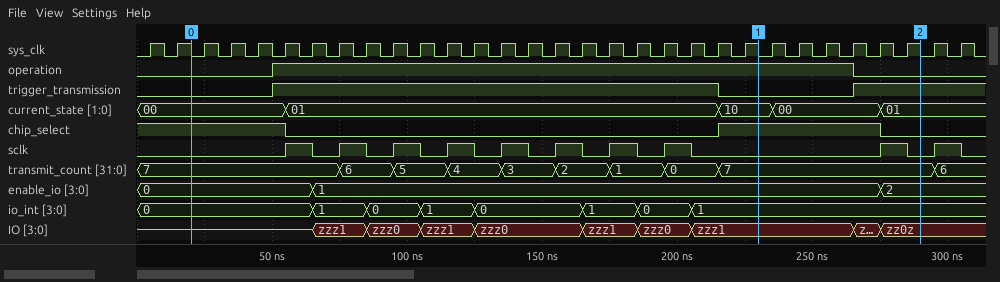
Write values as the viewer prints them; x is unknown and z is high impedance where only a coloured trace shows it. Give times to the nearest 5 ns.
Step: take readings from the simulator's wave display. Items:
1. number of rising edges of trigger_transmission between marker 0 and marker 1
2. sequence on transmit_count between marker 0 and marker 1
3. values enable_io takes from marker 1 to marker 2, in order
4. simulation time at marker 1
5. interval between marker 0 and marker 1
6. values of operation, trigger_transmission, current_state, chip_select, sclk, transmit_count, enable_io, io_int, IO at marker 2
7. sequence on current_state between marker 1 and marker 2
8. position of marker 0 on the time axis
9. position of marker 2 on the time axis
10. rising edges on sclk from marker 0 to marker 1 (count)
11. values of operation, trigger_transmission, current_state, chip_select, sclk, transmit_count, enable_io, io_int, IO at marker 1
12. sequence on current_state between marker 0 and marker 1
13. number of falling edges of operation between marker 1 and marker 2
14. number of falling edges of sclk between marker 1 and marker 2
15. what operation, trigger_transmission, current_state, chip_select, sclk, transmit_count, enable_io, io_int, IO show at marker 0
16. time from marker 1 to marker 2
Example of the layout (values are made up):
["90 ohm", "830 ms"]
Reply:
["1", "7, 6, 5, 4, 3, 2, 1, 0, 7", "1, 2", "230 ns", "210 ns", "operation=0, trigger_transmission=1, current_state=01, chip_select=0, sclk=0, transmit_count=7, enable_io=2, io_int=1, IO=zz0z", "10, 00, 01", "20 ns", "290 ns", "8", "operation=1, trigger_transmission=0, current_state=10, chip_select=1, sclk=0, transmit_count=7, enable_io=1, io_int=1, IO=zzz1", "00, 01, 10", "1", "1", "operation=0, trigger_transmission=0, current_state=00, chip_select=1, sclk=0, transmit_count=7, enable_io=0, io_int=0, IO=z", "60 ns"]
